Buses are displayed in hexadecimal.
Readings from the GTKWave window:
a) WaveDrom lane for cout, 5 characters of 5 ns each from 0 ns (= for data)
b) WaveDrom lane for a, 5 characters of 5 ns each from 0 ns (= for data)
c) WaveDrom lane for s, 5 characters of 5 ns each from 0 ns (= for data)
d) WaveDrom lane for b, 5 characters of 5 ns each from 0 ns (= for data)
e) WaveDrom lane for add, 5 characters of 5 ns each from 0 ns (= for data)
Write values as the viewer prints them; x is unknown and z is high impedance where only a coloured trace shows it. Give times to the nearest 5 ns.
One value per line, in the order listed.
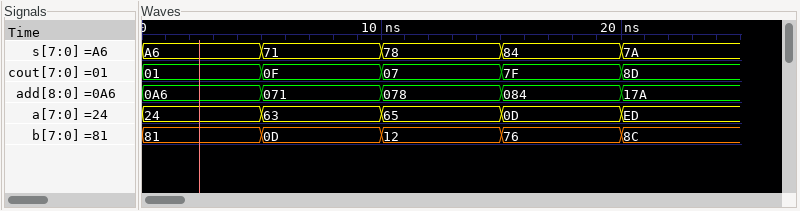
{name: 'cout', wave: '=====', data: '01 0F 07 7F 8D'}
{name: 'a', wave: '=====', data: '24 63 65 0D ED'}
{name: 's', wave: '=====', data: 'A6 71 78 84 7A'}
{name: 'b', wave: '=====', data: '81 0D 12 76 8C'}
{name: 'add', wave: '=====', data: '0A6 071 078 084 17A'}
